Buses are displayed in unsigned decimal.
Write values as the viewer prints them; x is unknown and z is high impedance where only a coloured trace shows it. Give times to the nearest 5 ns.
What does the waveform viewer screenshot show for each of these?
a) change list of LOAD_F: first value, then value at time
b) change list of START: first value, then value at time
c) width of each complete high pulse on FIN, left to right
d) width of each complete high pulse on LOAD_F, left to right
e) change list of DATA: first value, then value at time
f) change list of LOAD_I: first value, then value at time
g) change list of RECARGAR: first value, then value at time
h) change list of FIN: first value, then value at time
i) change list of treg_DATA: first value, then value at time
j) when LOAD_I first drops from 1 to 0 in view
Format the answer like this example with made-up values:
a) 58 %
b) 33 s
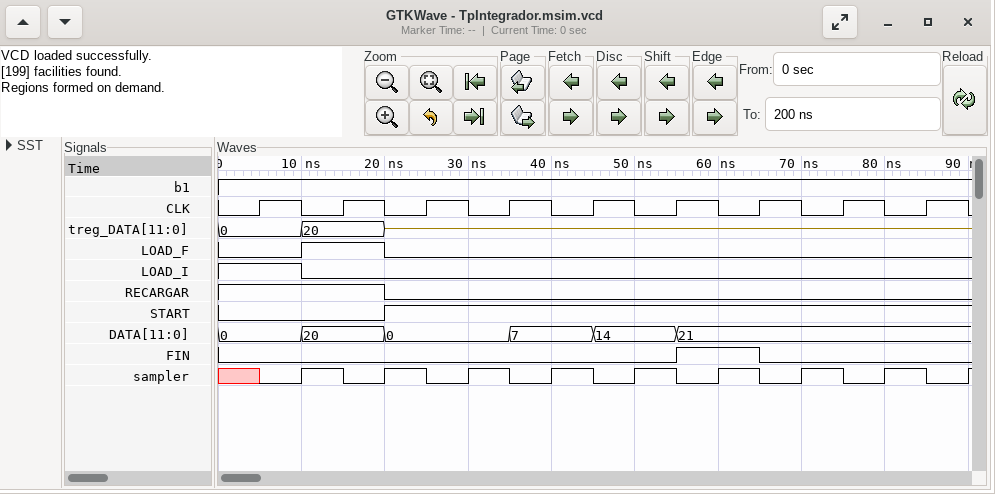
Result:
a) 0, 1 at 10 ns, 0 at 20 ns
b) 0, 1 at 20 ns
c) 10 ns
d) 10 ns
e) 0, 20 at 10 ns, 0 at 20 ns, 7 at 35 ns, 14 at 45 ns, 21 at 55 ns
f) 1, 0 at 10 ns
g) 1, 0 at 20 ns
h) 0, 1 at 55 ns, 0 at 65 ns
i) 0, 20 at 10 ns, z at 20 ns
j) 10 ns
